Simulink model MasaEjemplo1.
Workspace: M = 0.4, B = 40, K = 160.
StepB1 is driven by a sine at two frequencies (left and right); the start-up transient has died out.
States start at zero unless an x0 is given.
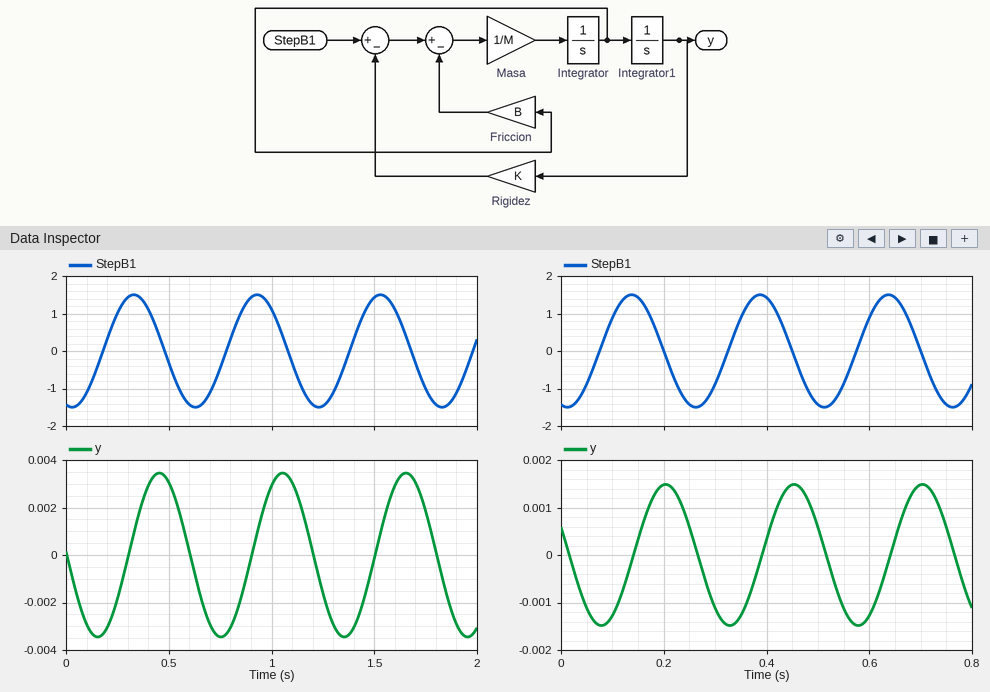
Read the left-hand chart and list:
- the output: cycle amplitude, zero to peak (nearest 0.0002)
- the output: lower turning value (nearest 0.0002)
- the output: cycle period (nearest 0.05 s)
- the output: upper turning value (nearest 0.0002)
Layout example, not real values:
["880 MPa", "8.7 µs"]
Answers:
["0.0034", "-0.0034", "0.60 s", "0.0034"]
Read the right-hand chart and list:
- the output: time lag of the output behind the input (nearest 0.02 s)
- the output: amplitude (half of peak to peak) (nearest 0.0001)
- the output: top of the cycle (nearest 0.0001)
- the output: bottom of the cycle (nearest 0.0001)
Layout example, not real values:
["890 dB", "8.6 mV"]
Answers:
["0.06 s", "0.0015", "0.0015", "-0.0015"]
